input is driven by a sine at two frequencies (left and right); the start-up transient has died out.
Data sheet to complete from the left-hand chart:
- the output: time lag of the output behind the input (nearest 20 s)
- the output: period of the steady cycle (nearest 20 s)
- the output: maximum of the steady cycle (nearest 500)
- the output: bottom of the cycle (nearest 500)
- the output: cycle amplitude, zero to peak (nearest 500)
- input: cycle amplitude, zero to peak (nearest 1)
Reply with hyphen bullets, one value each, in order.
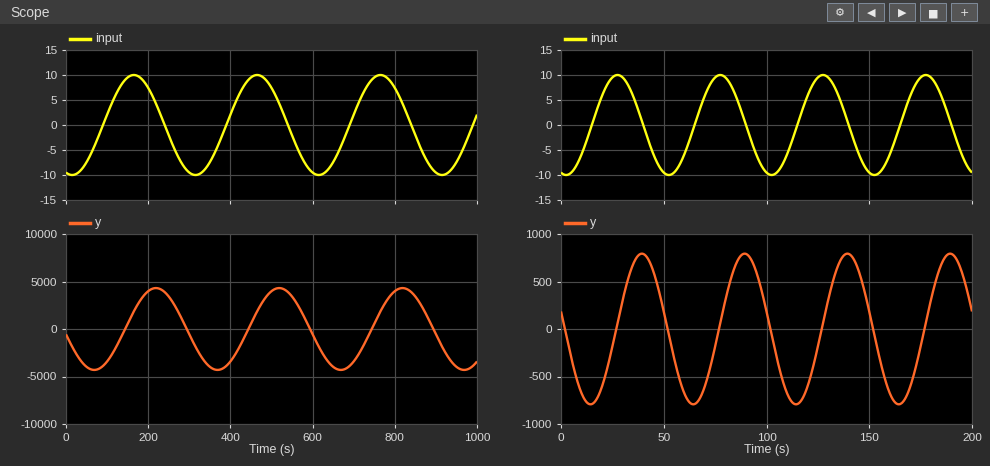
- 60 s
- 300 s
- 4500
- -4500
- 4500
- 10
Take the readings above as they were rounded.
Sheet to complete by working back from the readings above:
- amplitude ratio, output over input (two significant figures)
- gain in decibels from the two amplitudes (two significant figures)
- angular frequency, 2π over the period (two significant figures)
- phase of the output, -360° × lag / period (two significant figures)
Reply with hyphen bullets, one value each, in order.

- 450
- 53 dB
- 0.021 rad/s
- -72°
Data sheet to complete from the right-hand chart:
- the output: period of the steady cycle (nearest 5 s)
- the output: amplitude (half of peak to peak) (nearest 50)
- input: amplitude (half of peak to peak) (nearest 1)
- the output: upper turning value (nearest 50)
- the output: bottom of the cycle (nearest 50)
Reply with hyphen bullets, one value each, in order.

- 50 s
- 800
- 10
- 800
- -800
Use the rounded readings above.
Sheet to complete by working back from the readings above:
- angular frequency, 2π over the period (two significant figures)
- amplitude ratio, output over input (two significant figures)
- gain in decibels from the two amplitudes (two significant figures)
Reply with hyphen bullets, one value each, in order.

- 0.13 rad/s
- 80
- 38 dB
